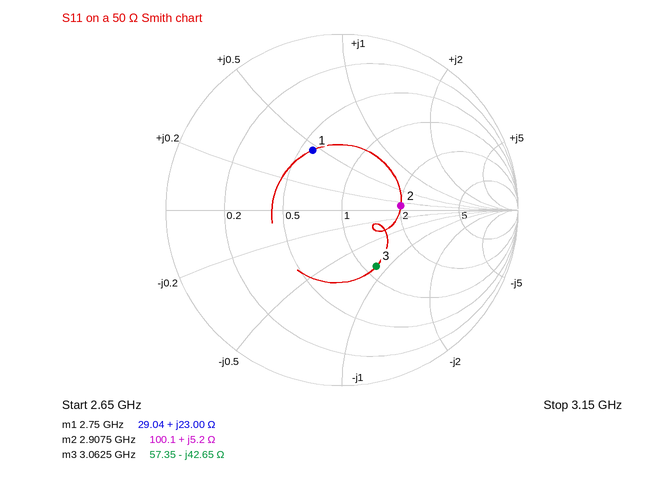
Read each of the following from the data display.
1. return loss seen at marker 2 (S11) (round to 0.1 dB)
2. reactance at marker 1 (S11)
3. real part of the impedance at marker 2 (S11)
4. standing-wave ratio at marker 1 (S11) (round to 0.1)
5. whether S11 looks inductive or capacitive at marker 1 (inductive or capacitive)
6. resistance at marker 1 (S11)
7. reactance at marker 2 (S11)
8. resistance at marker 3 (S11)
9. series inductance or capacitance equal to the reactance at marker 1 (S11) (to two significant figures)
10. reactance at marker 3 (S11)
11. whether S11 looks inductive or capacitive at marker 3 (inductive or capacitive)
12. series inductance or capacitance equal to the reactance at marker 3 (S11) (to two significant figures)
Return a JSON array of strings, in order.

["9.5 dB", "+23.00 Ω", "100.1 Ω", "2.2", "inductive", "29.04 Ω", "+5.2 Ω", "57.35 Ω", "1.3 nH", "-42.65 Ω", "capacitive", "1.2 pF"]
